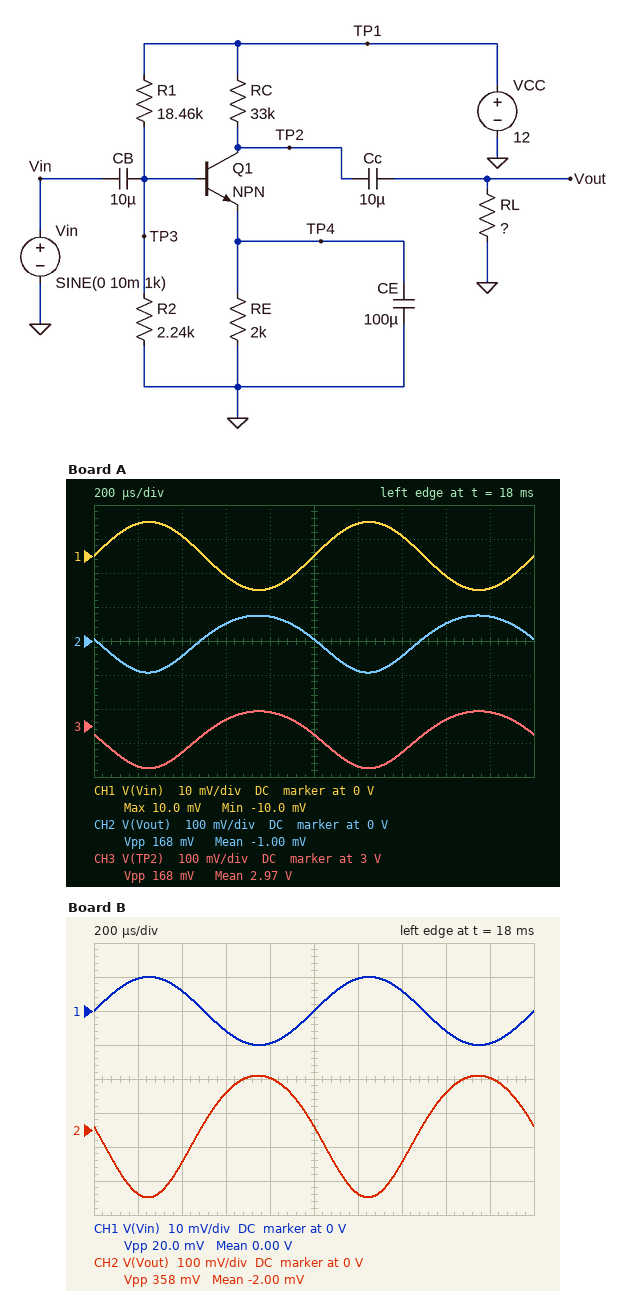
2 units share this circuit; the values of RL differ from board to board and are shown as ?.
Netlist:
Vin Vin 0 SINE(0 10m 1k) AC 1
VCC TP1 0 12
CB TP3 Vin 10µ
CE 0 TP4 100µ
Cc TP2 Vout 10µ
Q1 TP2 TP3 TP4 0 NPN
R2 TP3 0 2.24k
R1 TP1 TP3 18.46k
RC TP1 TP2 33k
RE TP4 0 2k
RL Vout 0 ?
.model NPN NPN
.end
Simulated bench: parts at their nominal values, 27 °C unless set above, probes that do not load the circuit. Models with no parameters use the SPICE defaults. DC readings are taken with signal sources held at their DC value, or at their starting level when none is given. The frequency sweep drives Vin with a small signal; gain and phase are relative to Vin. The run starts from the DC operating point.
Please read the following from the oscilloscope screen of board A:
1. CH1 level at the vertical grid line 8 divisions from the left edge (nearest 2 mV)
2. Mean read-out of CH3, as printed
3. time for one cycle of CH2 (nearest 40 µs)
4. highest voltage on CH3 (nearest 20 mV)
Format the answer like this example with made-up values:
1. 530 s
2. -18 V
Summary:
1. -6 mV
2. 2.97 V
3. 1.00 ms
4. 3.04 V
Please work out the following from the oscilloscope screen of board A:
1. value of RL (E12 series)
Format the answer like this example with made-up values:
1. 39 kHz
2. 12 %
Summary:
1. 820 Ω
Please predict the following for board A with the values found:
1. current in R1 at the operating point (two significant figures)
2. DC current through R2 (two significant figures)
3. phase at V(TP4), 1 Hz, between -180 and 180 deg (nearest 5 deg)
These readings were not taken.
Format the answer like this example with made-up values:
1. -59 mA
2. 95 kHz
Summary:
1. 580 µA
2. 580 µA
3. 80 deg
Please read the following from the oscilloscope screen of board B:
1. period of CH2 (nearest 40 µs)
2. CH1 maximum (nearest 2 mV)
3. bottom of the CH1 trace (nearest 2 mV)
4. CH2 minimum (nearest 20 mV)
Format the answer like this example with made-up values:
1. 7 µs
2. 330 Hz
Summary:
1. 1.00 ms
2. 10 mV
3. -10 mV
4. -200 mV
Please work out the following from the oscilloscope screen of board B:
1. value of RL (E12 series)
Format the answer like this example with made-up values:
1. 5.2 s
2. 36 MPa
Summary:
1. 1.8 kΩ
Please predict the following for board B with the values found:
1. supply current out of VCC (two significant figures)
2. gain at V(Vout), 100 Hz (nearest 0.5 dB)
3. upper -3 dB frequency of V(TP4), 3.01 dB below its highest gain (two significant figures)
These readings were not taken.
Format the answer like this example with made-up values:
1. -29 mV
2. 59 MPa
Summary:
1. 850 µA
2. 25.0 dB
3. 32 Hz
